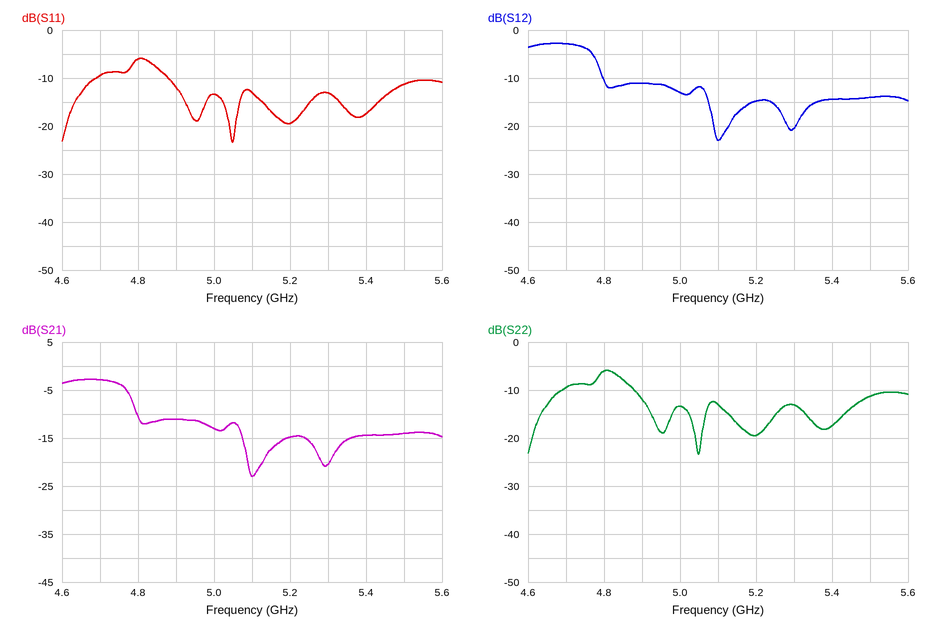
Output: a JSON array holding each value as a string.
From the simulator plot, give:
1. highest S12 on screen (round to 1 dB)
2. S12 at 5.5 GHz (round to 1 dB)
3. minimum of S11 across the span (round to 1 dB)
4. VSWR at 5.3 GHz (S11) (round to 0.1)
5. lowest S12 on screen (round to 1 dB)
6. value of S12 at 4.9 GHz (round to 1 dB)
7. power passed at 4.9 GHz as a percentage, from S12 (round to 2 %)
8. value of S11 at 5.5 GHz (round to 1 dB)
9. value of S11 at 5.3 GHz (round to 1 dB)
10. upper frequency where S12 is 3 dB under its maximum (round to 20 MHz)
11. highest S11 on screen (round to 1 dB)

["-3 dB", "-14 dB", "-23 dB", "1.6", "-23 dB", "-11 dB", "8 %", "-11 dB", "-13 dB", "4.78 GHz", "-6 dB"]
